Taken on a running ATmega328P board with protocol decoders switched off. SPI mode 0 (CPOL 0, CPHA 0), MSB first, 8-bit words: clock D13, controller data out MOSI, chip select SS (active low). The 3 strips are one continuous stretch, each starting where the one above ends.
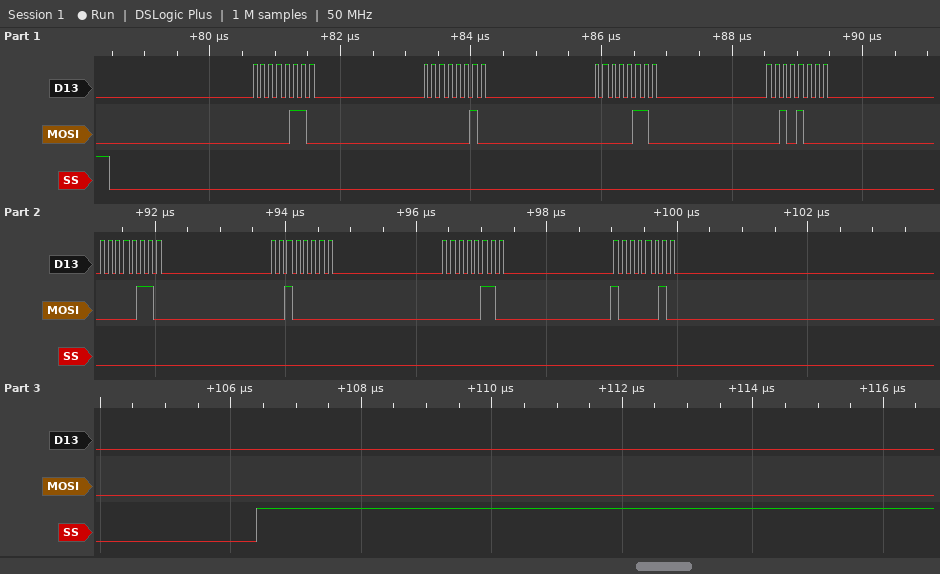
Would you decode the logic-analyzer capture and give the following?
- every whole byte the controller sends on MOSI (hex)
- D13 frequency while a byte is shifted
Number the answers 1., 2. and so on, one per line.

1. 06 02 06 28 06 20 06 82
2. 8 MHz
